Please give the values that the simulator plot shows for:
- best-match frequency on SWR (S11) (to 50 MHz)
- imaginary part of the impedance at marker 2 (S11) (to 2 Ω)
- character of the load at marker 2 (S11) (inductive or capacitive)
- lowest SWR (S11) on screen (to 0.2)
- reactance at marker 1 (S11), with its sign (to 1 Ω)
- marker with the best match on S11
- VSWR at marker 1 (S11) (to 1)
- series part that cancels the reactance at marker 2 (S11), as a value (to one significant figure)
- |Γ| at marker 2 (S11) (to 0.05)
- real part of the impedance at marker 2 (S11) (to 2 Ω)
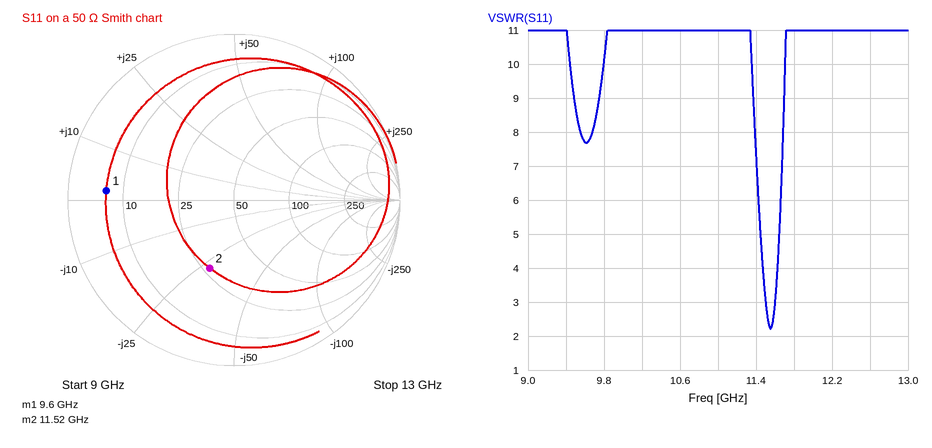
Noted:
11.55 GHz
-28 Ω
capacitive
2.2
+2 Ω
marker 2
8
400 pH
0.45
28 Ω
